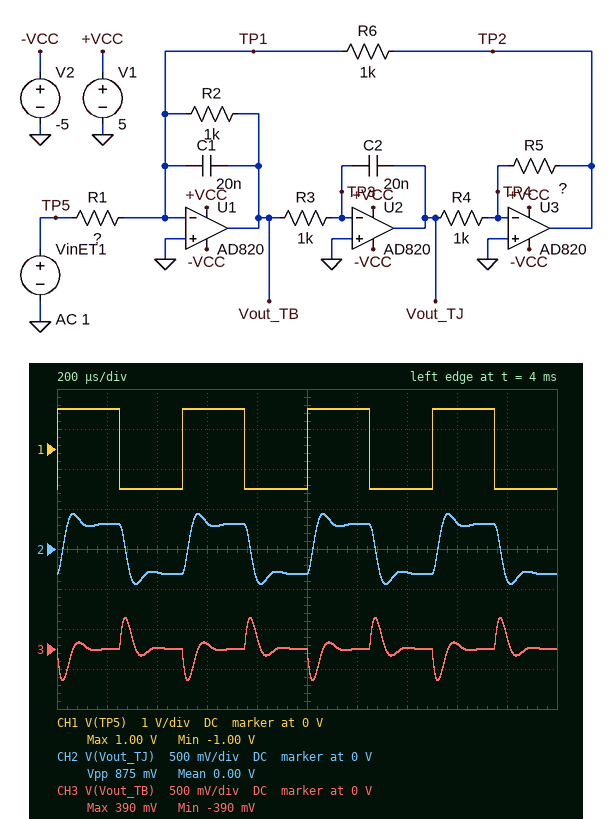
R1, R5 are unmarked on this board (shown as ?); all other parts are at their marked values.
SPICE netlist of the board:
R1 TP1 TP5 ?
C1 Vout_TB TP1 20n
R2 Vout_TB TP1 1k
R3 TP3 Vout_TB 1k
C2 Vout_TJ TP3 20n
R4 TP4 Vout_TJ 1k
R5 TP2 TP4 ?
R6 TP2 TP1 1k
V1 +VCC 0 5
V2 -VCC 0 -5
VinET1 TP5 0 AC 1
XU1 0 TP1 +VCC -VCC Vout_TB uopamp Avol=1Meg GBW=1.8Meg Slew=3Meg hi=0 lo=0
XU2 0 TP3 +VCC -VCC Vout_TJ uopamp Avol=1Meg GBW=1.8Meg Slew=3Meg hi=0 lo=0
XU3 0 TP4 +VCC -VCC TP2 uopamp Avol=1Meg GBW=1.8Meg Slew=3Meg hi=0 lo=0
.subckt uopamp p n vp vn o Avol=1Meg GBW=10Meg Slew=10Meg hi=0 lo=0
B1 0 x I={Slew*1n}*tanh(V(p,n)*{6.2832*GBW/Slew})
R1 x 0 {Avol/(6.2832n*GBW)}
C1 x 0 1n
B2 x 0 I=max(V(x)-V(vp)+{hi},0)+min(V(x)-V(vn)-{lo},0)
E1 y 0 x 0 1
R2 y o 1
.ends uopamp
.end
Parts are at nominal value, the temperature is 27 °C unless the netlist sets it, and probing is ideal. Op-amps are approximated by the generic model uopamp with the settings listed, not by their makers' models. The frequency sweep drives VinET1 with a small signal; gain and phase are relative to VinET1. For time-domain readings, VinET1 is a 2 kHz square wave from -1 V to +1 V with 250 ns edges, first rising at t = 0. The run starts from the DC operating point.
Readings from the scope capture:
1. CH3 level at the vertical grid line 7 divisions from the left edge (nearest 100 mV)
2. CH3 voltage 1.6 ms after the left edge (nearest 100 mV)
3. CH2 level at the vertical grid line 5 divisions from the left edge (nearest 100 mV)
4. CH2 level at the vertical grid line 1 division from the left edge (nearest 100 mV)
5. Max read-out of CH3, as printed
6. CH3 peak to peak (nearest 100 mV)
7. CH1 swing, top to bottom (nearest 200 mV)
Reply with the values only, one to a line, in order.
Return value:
0 V
100 mV
-300 mV
300 mV
390 mV
800 mV
2.0 V
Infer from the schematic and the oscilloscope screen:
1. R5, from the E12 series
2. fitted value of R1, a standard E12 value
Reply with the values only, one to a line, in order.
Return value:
1.2 kΩ
2.7 kΩ
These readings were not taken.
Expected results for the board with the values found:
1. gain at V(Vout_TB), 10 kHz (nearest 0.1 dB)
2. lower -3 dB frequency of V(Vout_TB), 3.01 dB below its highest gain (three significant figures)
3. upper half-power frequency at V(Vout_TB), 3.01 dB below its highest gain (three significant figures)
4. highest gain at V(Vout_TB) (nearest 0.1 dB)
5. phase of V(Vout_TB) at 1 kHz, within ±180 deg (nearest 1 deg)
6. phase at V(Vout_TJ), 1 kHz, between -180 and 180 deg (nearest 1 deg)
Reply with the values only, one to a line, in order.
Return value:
-8.9 dB
5.63 kHz
13.4 kHz
-8.4 dB
-96 deg
-6 deg
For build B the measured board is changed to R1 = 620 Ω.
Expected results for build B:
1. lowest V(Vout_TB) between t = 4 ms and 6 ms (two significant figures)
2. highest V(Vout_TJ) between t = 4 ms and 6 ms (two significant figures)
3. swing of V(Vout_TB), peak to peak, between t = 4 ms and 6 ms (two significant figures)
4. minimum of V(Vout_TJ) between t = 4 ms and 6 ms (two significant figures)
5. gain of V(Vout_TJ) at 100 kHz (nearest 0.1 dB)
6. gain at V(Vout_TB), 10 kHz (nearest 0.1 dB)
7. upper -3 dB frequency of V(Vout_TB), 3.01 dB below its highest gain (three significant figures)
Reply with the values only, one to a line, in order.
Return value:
-1.7 V
1.9 V
3.4 V
-1.9 V
-39.9 dB
3.9 dB
13.3 kHz
